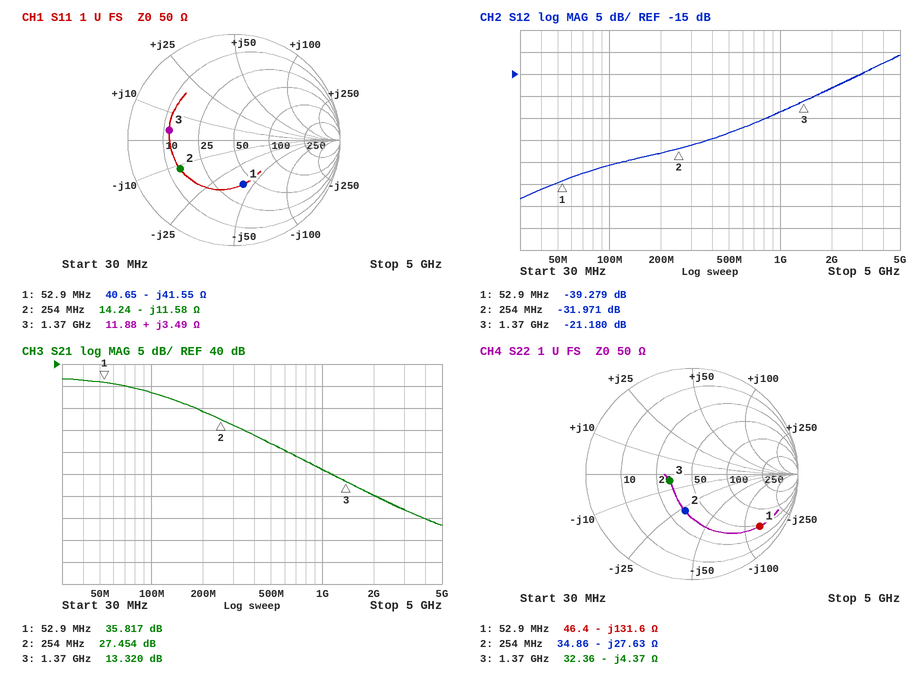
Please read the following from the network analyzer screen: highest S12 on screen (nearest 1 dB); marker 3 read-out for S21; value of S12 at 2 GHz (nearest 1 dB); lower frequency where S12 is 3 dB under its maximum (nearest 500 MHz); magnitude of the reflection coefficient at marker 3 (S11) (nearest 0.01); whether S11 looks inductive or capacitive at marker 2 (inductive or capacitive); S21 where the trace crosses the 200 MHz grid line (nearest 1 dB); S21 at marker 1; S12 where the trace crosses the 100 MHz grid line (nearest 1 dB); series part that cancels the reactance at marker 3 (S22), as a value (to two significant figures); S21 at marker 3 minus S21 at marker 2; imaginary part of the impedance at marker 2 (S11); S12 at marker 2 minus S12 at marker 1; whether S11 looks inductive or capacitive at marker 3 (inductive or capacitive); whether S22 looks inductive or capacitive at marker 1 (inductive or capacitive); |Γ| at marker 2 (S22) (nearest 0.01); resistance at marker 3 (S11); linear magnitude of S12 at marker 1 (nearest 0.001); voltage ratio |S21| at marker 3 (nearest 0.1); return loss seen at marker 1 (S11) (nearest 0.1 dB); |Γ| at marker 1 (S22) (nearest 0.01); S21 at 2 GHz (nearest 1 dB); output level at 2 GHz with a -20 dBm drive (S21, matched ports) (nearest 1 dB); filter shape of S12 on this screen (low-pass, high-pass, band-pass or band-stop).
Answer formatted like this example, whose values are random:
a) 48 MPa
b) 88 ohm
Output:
a) -11 dB
b) 13.320 dB
c) -18 dB
d) 3.5 GHz
e) 0.62
f) capacitive
g) 29 dB
h) 35.817 dB
i) -36 dB
j) 510 pH
k) -14.134 dB
l) -11.58 Ω
m) 7.308 dB
n) inductive
o) capacitive
p) 0.35
q) 11.88 Ω
r) 0.011
s) 4.6
t) 7.4 dB
u) 0.81
v) 10 dB
w) -10 dBm
x) high-pass
